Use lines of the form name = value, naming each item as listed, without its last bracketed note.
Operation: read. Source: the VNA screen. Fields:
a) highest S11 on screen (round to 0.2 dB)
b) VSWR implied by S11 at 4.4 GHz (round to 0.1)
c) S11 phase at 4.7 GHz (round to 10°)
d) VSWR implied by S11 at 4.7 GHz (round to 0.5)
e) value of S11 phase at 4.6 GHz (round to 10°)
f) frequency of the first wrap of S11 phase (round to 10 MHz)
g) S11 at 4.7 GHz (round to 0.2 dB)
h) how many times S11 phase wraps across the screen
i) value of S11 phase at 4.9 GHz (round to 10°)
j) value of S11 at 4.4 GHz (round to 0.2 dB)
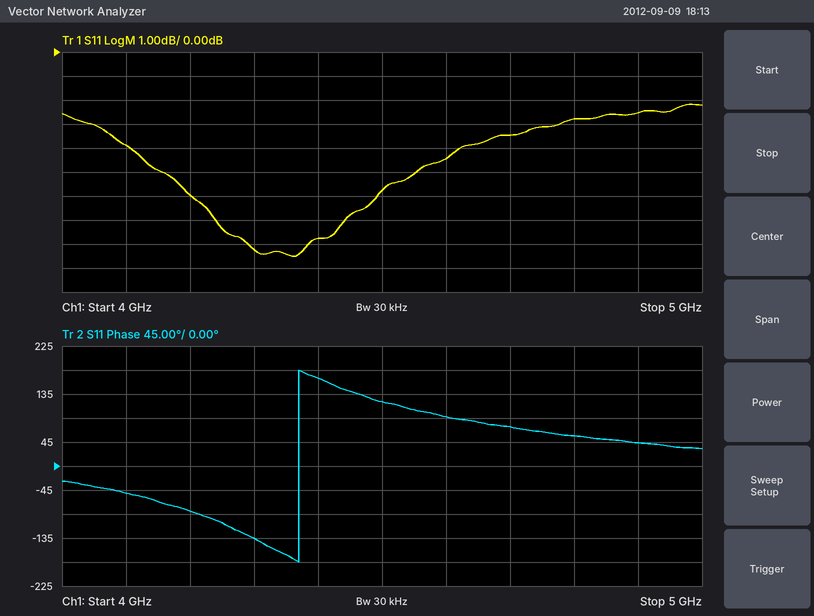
highest S11 on screen = -2.2 dB
VSWR implied by S11 at 4.4 GHz = 2.4
S11 phase at 4.7 GHz = 70°
VSWR implied by S11 at 4.7 GHz = 5.0
value of S11 phase at 4.6 GHz = 90°
frequency of the first wrap of S11 phase = 4.37 GHz
S11 at 4.7 GHz = -3.4 dB
how many times S11 phase wraps across the screen = 1
value of S11 phase at 4.9 GHz = 40°
value of S11 at 4.4 GHz = -7.8 dB
